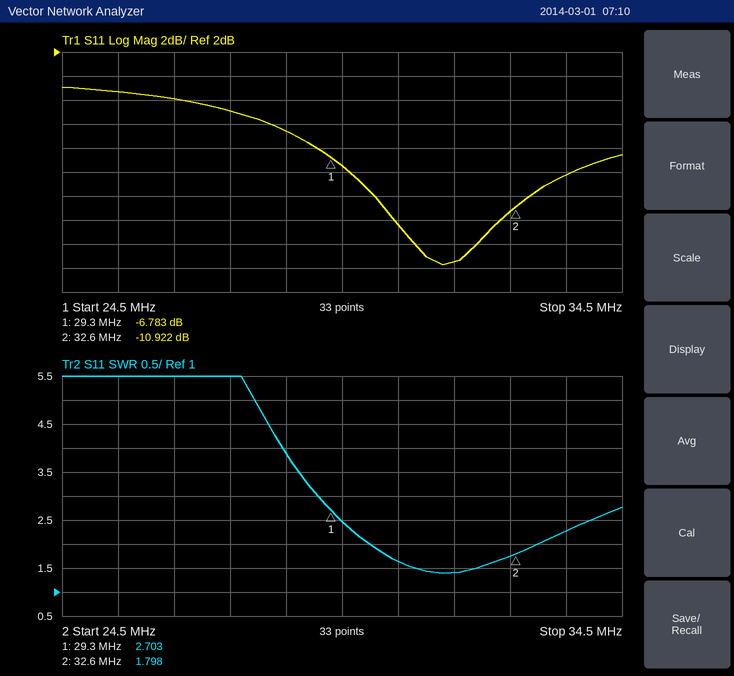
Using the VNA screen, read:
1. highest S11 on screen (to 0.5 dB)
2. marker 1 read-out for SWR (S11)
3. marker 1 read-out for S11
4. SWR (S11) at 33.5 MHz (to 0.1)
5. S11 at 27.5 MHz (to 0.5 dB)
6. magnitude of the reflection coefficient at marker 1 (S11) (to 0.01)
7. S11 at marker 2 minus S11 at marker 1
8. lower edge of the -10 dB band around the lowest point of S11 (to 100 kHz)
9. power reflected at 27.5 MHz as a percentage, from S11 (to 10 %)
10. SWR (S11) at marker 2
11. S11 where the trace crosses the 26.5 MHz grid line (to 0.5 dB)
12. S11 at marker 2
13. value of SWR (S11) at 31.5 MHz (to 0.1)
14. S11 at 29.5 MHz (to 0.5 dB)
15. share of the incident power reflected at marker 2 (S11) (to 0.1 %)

-1.0 dB
2.703
-6.783 dB
2.3
-3.0 dB
0.46
-4.139 dB
30.1 MHz
50 %
1.798
-2.0 dB
-10.922 dB
1.4
-7.5 dB
8.1 %
